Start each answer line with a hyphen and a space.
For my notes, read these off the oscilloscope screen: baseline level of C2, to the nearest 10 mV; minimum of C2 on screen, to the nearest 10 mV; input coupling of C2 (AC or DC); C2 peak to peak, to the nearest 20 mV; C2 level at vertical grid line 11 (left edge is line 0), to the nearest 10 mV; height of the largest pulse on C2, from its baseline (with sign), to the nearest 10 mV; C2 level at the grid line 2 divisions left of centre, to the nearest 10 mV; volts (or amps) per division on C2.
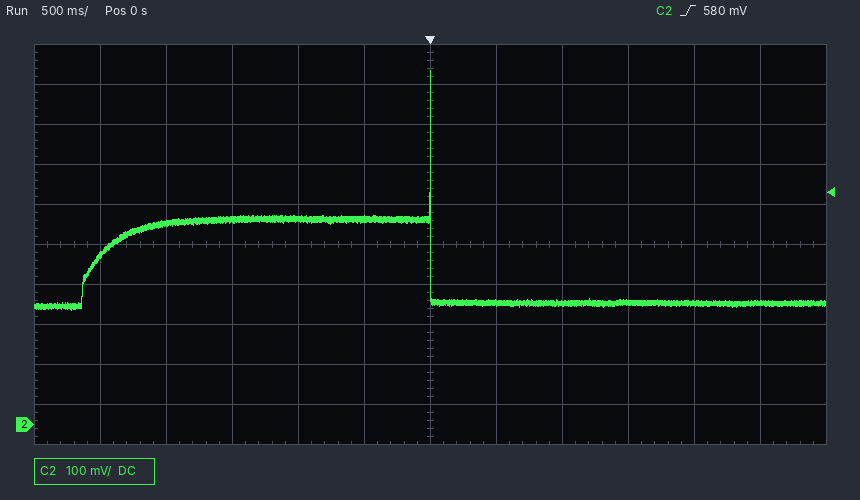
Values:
- 300 mV
- 290 mV
- DC
- 600 mV
- 300 mV
- +580 mV
- 510 mV
- 100 mV
